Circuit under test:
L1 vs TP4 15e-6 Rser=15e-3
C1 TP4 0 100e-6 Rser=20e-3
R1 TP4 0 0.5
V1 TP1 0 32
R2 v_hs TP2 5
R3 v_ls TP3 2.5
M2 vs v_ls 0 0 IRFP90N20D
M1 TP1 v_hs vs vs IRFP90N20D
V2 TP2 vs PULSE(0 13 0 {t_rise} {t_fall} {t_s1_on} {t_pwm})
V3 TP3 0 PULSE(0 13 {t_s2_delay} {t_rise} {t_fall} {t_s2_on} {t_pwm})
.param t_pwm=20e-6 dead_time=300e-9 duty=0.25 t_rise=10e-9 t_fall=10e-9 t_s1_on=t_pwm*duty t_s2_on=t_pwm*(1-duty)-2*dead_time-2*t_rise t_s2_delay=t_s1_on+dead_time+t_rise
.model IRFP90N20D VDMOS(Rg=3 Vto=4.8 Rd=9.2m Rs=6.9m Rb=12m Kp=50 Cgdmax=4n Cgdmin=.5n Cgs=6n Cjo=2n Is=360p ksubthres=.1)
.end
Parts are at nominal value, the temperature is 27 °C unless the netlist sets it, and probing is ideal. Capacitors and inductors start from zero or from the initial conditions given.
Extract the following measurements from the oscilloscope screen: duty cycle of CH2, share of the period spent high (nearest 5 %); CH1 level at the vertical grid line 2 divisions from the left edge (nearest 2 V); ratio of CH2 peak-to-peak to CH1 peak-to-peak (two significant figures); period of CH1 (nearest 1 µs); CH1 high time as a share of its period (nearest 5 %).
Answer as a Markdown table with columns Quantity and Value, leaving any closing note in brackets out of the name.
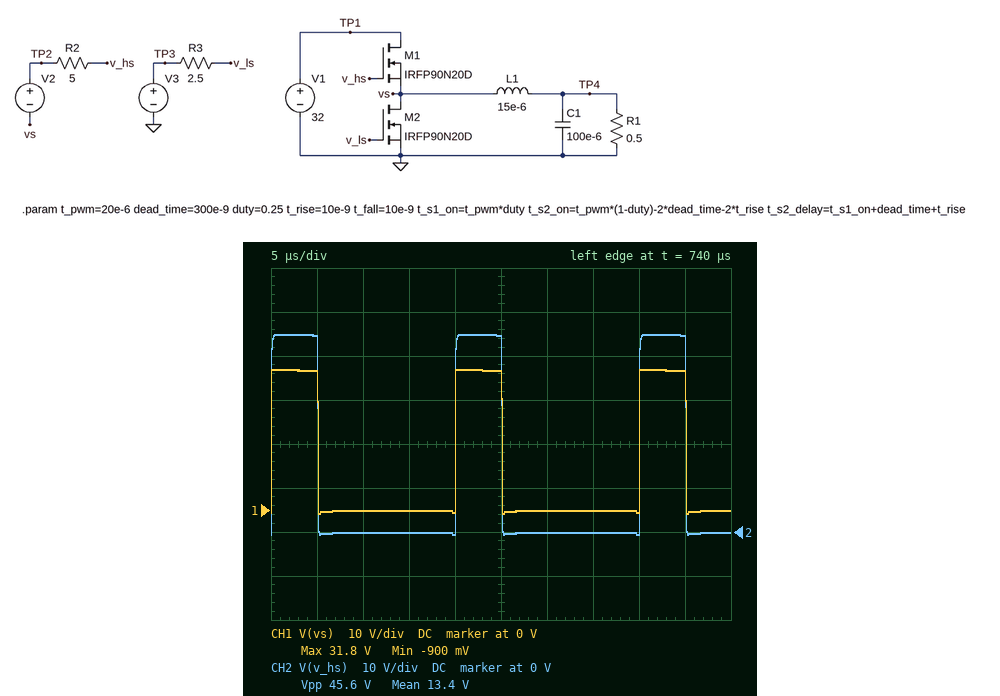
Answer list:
| Quantity | Value |
|---|---|
| duty cycle of CH2, share of the period spent high | 25 % |
| CH1 level at the vertical grid line 2 divisions from the left edge | 0 V |
| ratio of CH2 peak-to-peak to CH1 peak-to-peak | 1.4 |
| period of CH1 | 20 µs |
| CH1 high time as a share of its period | 25 % |
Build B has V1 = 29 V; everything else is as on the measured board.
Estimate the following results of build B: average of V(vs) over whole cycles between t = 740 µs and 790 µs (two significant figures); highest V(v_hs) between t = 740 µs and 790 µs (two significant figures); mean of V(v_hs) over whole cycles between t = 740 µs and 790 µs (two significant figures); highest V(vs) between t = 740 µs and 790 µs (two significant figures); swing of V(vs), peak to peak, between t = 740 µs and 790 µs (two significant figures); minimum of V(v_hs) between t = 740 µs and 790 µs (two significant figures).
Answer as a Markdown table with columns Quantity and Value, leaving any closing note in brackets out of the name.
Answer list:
| Quantity | Value |
|---|---|
| average of V(vs) over whole cycles between t = 740 µs and 790 µs | 7.1 V |
| highest V(v_hs) between t = 740 µs and 790 µs | 42 V |
| mean of V(v_hs) over whole cycles between t = 740 µs and 790 µs | 10 V |
| highest V(vs) between t = 740 µs and 790 µs | 29 V |
| swing of V(vs), peak to peak, between t = 740 µs and 790 µs | 30 V |
| minimum of V(v_hs) between t = 740 µs and 790 µs | -760 mV |
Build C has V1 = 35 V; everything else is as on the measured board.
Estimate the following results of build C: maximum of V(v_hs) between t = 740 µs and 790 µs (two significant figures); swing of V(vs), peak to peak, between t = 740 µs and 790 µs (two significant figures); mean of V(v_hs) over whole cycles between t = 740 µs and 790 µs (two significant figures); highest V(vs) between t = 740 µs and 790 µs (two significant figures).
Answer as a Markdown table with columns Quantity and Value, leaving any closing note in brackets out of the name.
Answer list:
| Quantity | Value |
|---|---|
| maximum of V(v_hs) between t = 740 µs and 790 µs | 48 V |
| swing of V(vs), peak to peak, between t = 740 µs and 790 µs | 36 V |
| mean of V(v_hs) over whole cycles between t = 740 µs and 790 µs | 12 V |
| highest V(vs) between t = 740 µs and 790 µs | 35 V |
